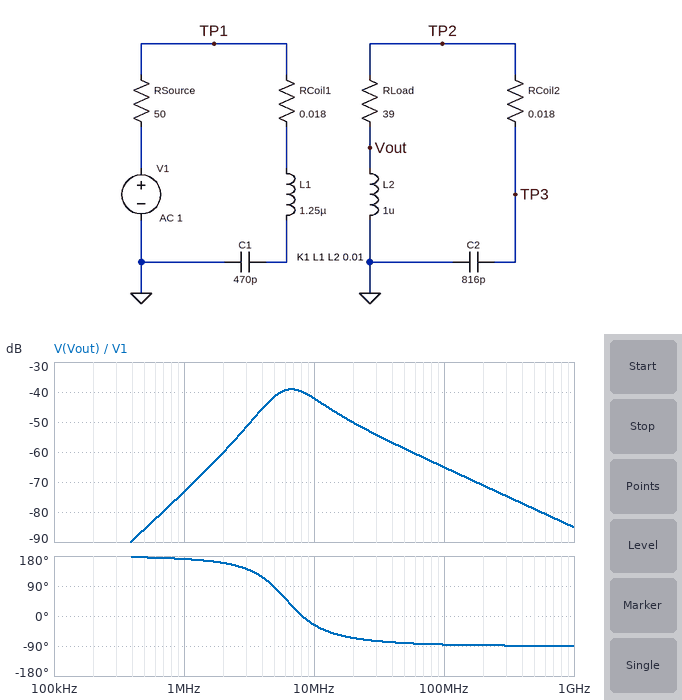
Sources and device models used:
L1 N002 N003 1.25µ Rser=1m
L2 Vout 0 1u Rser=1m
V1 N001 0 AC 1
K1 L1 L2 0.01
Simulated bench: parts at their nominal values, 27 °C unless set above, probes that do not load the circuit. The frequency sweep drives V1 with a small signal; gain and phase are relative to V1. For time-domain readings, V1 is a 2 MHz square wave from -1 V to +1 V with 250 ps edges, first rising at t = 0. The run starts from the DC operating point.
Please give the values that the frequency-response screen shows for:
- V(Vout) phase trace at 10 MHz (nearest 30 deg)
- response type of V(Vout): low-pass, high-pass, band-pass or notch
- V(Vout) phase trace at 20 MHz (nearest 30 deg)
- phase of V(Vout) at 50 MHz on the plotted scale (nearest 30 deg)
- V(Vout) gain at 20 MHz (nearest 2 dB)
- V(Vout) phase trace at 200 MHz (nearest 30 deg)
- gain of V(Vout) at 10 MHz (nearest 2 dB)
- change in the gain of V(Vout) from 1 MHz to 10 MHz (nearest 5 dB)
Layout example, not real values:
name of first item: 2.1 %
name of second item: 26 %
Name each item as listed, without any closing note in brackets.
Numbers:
V(Vout) phase trace at 10 MHz: -30 deg
response type of V(Vout): low-pass, high-pass, band-pass or notch: band-pass
V(Vout) phase trace at 20 MHz: -60 deg
phase of V(Vout) at 50 MHz on the plotted scale: -90 deg
V(Vout) gain at 20 MHz: -50 dB
V(Vout) phase trace at 200 MHz: -90 deg
gain of V(Vout) at 10 MHz: -42 dB
change in the gain of V(Vout) from 1 MHz to 10 MHz: 30 dB
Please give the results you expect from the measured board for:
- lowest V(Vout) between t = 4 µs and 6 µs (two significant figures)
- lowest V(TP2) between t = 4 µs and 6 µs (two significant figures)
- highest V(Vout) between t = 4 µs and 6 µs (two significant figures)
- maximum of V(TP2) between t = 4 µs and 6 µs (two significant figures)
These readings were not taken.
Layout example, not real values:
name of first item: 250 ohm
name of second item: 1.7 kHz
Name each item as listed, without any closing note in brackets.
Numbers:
lowest V(Vout) between t = 4 µs and 6 µs: -7.7 mV
lowest V(TP2) between t = 4 µs and 6 µs: -4.3 mV
highest V(Vout) between t = 4 µs and 6 µs: 7.7 mV
maximum of V(TP2) between t = 4 µs and 6 µs: 4.3 mV
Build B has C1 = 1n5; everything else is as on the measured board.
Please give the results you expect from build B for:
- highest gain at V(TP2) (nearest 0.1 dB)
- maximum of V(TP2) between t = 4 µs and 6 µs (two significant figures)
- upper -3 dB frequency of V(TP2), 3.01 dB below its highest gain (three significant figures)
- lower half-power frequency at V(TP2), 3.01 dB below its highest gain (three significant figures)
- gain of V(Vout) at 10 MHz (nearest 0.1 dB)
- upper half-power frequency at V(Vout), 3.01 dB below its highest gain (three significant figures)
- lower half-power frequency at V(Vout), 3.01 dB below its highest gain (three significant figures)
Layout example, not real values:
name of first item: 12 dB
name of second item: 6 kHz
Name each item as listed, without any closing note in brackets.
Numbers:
highest gain at V(TP2): -43.8 dB
maximum of V(TP2) between t = 4 µs and 6 µs: 5.2 mV
upper -3 dB frequency of V(TP2), 3.01 dB below its highest gain: 7.52 MHz
lower half-power frequency at V(TP2), 3.01 dB below its highest gain: 3.09 MHz
gain of V(Vout) at 10 MHz: -44.1 dB
upper half-power frequency at V(Vout), 3.01 dB below its highest gain: 9.40 MHz
lower half-power frequency at V(Vout), 3.01 dB below its highest gain: 3.58 MHz
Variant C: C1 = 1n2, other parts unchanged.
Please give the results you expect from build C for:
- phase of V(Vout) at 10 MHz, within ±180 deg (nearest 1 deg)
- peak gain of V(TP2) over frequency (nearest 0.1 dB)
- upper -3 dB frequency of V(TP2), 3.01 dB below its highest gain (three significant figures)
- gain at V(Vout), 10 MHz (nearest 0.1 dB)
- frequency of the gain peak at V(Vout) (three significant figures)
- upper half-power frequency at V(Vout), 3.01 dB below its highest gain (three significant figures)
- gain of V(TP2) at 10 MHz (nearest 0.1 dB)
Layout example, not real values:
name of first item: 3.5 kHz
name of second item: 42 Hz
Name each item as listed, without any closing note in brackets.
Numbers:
phase of V(Vout) at 10 MHz, within ±180 deg: -37 deg
peak gain of V(TP2) over frequency: -43.5 dB
upper -3 dB frequency of V(TP2), 3.01 dB below its highest gain: 7.54 MHz
gain at V(Vout), 10 MHz: -43.9 dB
frequency of the gain peak at V(Vout): 5.70 MHz
upper half-power frequency at V(Vout), 3.01 dB below its highest gain: 9.33 MHz
gain of V(TP2) at 10 MHz: -50.9 dB
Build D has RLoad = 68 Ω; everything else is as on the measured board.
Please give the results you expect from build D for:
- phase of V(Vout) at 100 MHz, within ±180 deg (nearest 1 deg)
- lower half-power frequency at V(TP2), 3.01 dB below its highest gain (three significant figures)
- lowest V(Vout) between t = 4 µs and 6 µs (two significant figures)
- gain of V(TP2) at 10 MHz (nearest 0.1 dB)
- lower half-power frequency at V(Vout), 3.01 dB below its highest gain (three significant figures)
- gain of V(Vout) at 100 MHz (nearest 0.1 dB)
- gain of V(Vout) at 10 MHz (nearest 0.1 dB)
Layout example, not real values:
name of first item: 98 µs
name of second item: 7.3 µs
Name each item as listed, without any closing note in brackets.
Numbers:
phase of V(Vout) at 100 MHz, within ±180 deg: -82 deg
lower half-power frequency at V(TP2), 3.01 dB below its highest gain: 4.22 MHz
lowest V(Vout) between t = 4 µs and 6 µs: -8.7 mV
gain of V(TP2) at 10 MHz: -51.9 dB
lower half-power frequency at V(Vout), 3.01 dB below its highest gain: 5.14 MHz
gain of V(Vout) at 100 MHz: -60.3 dB
gain of V(Vout) at 10 MHz: -40.7 dB
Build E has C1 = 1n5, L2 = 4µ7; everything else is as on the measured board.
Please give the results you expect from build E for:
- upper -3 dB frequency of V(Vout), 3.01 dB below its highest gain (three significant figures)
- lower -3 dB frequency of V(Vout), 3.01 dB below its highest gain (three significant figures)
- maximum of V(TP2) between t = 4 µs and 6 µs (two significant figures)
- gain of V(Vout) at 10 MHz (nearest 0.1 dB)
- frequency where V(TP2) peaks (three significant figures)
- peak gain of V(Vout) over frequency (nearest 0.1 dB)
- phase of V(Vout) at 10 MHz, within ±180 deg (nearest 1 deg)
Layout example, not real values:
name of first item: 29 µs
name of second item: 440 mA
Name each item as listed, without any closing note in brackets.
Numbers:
upper -3 dB frequency of V(Vout), 3.01 dB below its highest gain: 3.59 MHz
lower -3 dB frequency of V(Vout), 3.01 dB below its highest gain: 2.14 MHz
maximum of V(TP2) between t = 4 µs and 6 µs: 10 mV
gain of V(Vout) at 10 MHz: -51.0 dB
frequency where V(TP2) peaks: 2.64 MHz
peak gain of V(Vout) over frequency: -35.9 dB
phase of V(Vout) at 10 MHz, within ±180 deg: -72 deg
